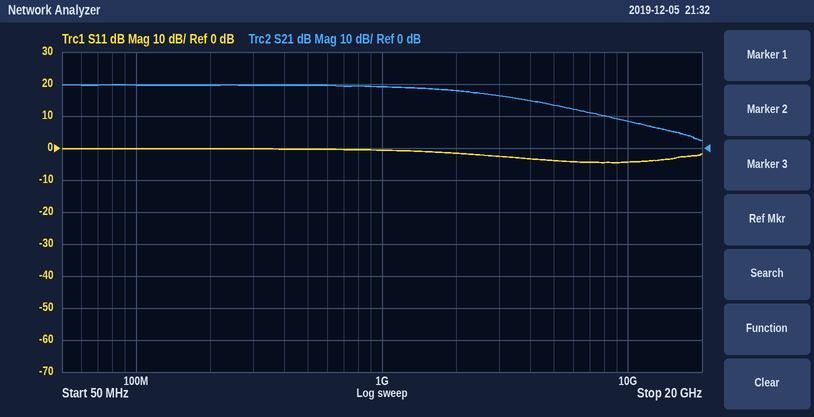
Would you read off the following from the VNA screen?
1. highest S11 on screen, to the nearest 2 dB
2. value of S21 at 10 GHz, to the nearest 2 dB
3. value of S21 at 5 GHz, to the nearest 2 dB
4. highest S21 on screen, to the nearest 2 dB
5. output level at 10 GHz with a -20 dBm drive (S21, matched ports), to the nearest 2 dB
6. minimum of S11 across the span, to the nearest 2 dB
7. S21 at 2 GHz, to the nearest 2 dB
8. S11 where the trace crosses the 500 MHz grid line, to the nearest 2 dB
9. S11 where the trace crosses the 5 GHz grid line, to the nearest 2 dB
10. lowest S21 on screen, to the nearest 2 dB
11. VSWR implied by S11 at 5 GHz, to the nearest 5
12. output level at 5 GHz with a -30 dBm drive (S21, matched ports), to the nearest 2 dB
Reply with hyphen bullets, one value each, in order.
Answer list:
- 0 dB
- 8 dB
- 14 dB
- 20 dB
- -12 dBm
- -4 dB
- 18 dB
- 0 dB
- -4 dB
- 2 dB
- 5
- -16 dBm
